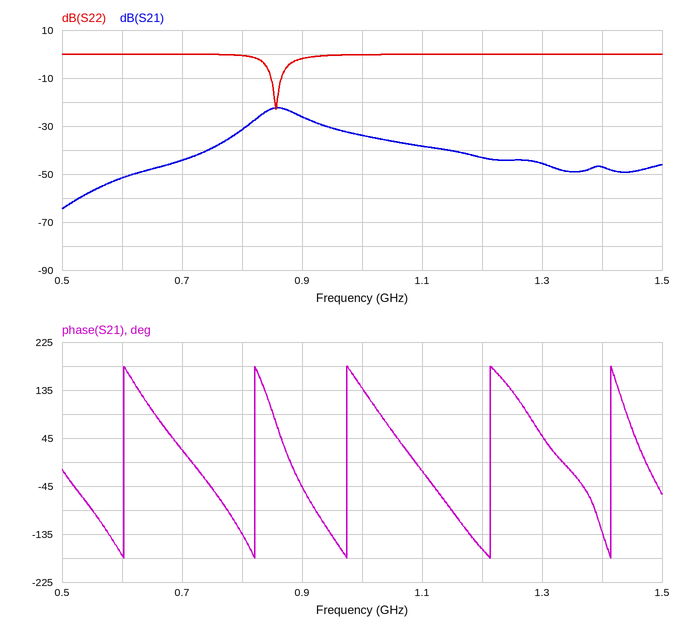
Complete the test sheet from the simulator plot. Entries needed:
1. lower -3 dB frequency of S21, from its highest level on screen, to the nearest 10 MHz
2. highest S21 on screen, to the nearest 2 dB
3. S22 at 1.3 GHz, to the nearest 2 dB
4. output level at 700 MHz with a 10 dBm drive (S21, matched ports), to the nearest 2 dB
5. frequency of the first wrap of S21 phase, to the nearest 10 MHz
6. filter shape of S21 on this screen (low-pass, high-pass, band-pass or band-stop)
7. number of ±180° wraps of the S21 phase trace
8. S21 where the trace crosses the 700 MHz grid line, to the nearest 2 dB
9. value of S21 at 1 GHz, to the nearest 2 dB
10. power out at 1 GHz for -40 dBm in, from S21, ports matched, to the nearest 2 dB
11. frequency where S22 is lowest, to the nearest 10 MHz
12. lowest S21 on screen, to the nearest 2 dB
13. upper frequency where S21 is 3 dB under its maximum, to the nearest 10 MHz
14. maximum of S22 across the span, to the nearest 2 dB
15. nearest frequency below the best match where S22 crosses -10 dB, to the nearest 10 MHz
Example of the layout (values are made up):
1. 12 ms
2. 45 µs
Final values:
1. 830 MHz
2. -22 dB
3. 0 dB
4. -34 dBm
5. 600 MHz
6. band-pass
7. 5
8. -44 dB
9. -34 dB
10. -74 dBm
11. 860 MHz
12. -64 dB
13. 890 MHz
14. 0 dB
15. 850 MHz
